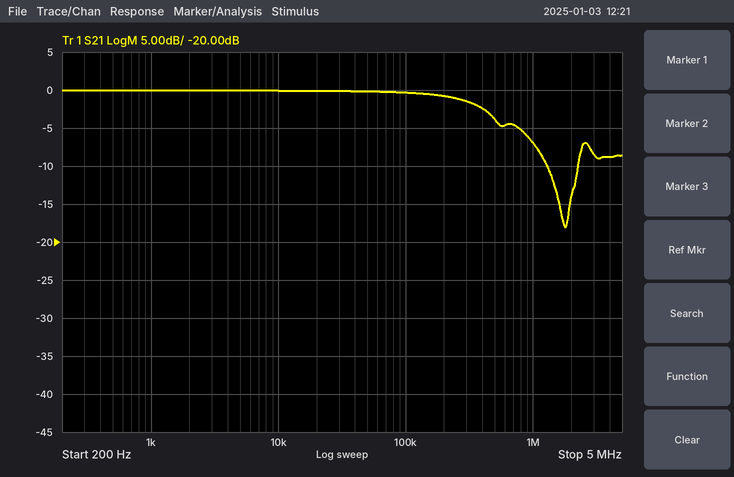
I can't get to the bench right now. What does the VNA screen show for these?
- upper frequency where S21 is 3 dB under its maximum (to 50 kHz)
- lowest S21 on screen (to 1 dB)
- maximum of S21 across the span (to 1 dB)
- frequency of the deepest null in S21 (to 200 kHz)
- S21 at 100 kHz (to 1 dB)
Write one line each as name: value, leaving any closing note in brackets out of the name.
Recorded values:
upper frequency where S21 is 3 dB under its maximum: 450 kHz
lowest S21 on screen: -18 dB
maximum of S21 across the span: 0 dB
frequency of the deepest null in S21: 1.8 MHz
S21 at 100 kHz: 0 dB
